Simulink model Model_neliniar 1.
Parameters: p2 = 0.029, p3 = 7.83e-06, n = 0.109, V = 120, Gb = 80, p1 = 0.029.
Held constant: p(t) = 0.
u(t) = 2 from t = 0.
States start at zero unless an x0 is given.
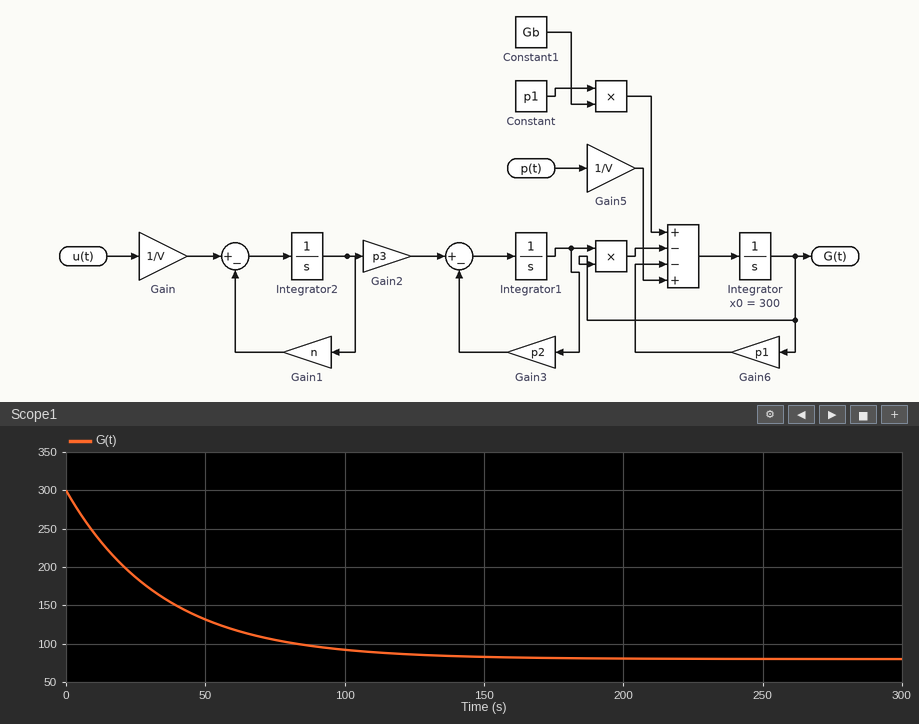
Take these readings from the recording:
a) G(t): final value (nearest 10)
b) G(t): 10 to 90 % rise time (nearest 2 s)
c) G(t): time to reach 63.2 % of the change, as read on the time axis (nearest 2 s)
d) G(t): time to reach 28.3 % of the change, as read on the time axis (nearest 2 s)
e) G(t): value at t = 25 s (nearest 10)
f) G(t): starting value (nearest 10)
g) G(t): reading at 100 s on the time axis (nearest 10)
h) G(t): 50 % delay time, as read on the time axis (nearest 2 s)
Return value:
80
76 s
34 s
12 s
190
300
90
24 s
